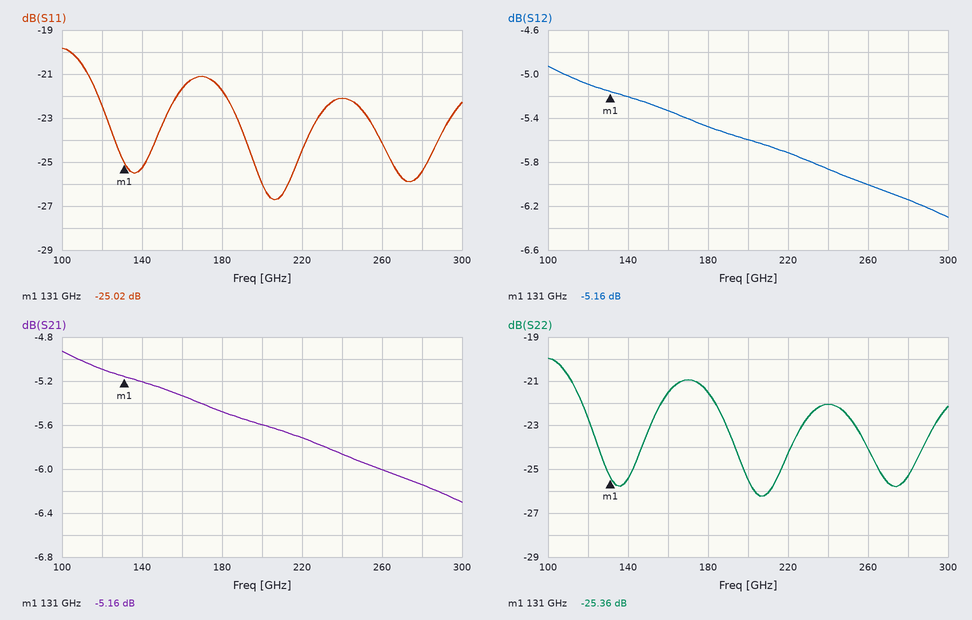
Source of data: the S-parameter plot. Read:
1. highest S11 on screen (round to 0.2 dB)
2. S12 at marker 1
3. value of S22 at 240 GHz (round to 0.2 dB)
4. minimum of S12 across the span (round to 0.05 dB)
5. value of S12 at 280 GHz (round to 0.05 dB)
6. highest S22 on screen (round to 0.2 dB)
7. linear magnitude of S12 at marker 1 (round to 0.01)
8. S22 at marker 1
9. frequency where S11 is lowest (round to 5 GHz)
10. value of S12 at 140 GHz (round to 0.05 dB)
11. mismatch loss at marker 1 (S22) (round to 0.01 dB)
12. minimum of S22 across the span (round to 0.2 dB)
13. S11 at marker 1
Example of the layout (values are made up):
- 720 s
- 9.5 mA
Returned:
- -19.8 dB
- -5.16 dB
- -22.0 dB
- -6.30 dB
- -6.15 dB
- -20.0 dB
- 0.55
- -25.36 dB
- 205 GHz
- -5.20 dB
- 0.01 dB
- -26.2 dB
- -25.02 dB
